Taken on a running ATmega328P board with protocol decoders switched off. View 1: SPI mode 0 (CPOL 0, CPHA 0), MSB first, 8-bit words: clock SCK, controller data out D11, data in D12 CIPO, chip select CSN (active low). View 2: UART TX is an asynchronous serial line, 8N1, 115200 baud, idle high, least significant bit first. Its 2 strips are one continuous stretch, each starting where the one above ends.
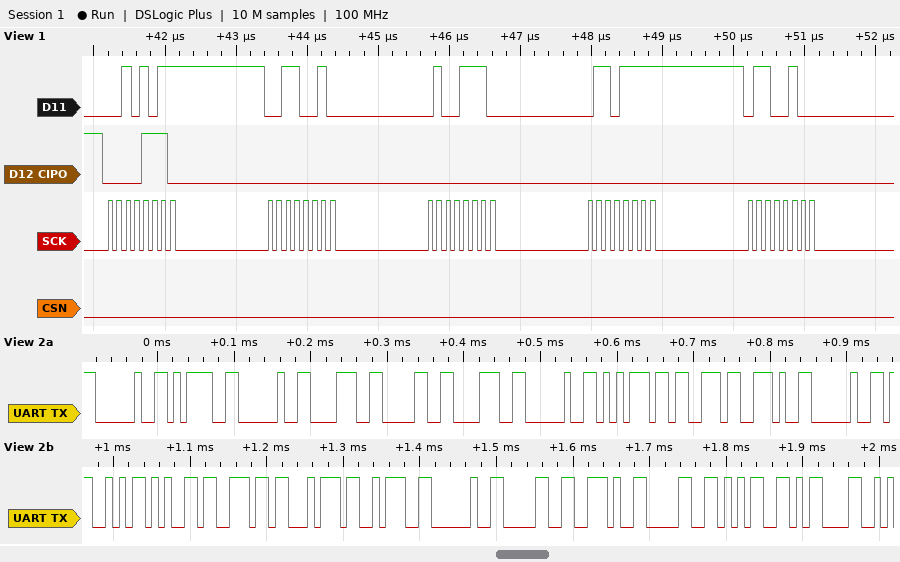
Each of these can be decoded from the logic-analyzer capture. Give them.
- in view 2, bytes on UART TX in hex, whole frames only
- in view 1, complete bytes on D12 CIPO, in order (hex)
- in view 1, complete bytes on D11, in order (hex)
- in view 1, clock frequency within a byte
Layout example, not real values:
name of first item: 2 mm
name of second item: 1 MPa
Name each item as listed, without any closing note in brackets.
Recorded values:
in view 2, bytes on UART TX in hex, whole frames only: 0x20 0x3D 0x20 0x38 0x30 0x38 0x20 0x75 0x73 0x2E 0x20 0x53 0x65 0x6E 0x74 0x3A 0x20 0x30 0x2E 0x30 0x35 0x0D
in view 1, complete bytes on D12 CIPO, in order: 0E 00 00 00 00
in view 1, complete bytes on D11, in order: 2B 32 4E 6F 64
in view 1, clock frequency within a byte: 8 MHz
